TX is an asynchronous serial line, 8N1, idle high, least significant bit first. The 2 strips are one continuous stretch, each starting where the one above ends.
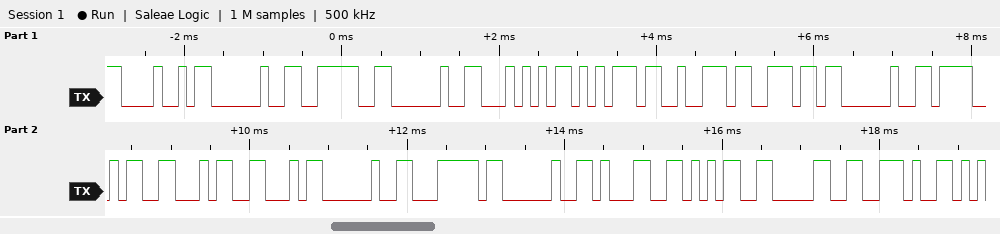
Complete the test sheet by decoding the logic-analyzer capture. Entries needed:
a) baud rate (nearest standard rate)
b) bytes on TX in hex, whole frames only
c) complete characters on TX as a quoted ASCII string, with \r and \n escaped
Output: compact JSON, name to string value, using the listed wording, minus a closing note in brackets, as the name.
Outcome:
{"baud rate": "9600 baud", "bytes on TX in hex, whole frames only": "0x48 0x20 0x3E 0x20 0x54 0x75 0x72 0x6E 0x20 0x4F 0x46 0x46 0x20 0x7C 0x20 0x31 0x35 0x30 0x2E", "complete characters on TX as a quoted ASCII string, with \\r and \\n escaped": "\"H > Turn OFF | 150.\""}
